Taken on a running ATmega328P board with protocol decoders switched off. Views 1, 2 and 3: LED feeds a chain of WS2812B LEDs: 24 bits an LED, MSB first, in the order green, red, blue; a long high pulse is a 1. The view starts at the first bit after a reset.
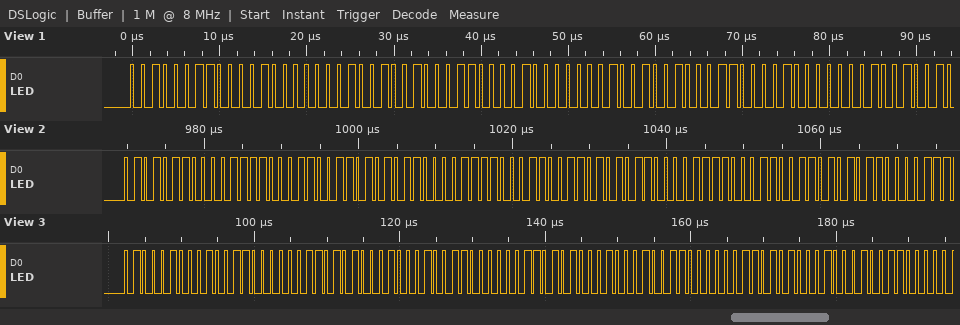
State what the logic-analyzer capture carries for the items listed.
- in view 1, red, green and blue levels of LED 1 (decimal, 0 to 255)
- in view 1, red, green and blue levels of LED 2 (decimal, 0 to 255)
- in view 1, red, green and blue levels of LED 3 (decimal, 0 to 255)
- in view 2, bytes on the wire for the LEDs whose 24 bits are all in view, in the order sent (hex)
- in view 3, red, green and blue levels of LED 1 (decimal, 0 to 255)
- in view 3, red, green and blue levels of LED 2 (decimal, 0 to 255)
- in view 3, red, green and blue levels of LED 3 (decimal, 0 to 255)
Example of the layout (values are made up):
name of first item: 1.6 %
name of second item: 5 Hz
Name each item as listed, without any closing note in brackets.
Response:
in view 1, red, green and blue levels of LED 1: 8, 35, 9
in view 1, red, green and blue levels of LED 2: 8, 35, 9
in view 1, red, green and blue levels of LED 3: 8, 35, 9
in view 2, bytes on the wire for the LEDs whose 24 bits are all in view, in the order sent: 56 1E 33 56 1E 33 56 1E 33
in view 3, red, green and blue levels of LED 1: 76, 68, 13
in view 3, red, green and blue levels of LED 2: 76, 68, 13
in view 3, red, green and blue levels of LED 3: 76, 68, 13
